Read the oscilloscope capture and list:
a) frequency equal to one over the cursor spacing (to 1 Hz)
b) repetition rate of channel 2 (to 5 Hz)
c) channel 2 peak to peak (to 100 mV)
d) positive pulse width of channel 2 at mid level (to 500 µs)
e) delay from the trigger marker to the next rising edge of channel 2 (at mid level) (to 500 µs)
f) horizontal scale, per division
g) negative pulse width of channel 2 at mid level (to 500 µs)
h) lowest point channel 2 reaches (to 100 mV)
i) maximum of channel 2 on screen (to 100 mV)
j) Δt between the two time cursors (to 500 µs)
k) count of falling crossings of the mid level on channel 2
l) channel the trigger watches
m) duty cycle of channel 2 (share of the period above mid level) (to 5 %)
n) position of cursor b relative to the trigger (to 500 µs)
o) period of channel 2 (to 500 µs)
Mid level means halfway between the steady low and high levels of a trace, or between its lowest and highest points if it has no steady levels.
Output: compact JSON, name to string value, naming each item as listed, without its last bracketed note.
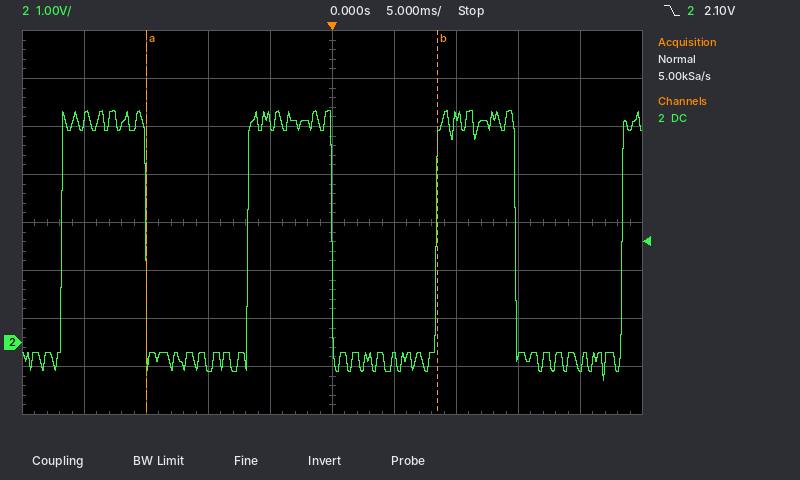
{"frequency equal to one over the cursor spacing": "43 Hz", "repetition rate of channel 2": "65 Hz", "channel 2 peak to peak": "5.6 V", "positive pulse width of channel 2 at mid level": "6.5 ms", "delay from the trigger marker to the next rising edge of channel 2 (at mid level)": "8.5 ms", "horizontal scale, per division": "5 ms", "negative pulse width of channel 2 at mid level": "8.5 ms", "lowest point channel 2 reaches": "-800 mV", "maximum of channel 2 on screen": "4.8 V", "Δt between the two time cursors": "23.5 ms", "count of falling crossings of the mid level on channel 2": "3", "channel the trigger watches": "channel 2", "duty cycle of channel 2 (share of the period above mid level)": "45 %", "position of cursor b relative to the trigger": "+8.5 ms", "period of channel 2": "15.0 ms"}
